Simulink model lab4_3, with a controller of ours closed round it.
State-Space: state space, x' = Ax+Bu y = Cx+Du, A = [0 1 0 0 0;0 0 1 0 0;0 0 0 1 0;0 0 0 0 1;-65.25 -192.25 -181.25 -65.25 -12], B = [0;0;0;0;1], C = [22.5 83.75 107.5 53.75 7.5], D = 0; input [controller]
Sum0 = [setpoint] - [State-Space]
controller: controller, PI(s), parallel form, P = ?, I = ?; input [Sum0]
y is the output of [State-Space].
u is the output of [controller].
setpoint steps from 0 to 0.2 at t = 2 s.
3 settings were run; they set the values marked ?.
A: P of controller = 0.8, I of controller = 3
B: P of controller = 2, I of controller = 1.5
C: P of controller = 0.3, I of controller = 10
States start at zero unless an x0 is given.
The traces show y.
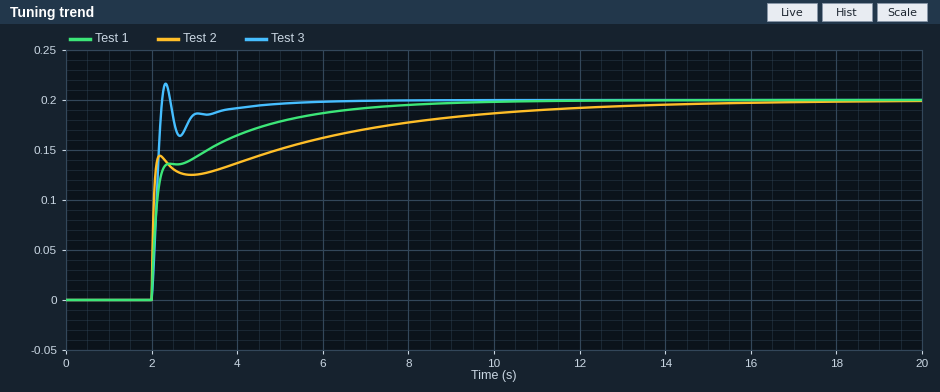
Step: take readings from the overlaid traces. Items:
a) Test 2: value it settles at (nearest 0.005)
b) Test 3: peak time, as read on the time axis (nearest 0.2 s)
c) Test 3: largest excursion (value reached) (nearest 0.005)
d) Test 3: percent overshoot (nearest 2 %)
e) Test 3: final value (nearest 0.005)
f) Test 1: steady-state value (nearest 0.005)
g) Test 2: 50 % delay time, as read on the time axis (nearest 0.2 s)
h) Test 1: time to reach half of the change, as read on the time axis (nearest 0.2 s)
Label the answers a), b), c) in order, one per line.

a) 0.200
b) 2.4 s
c) 0.215
d) 8 %
e) 0.200
f) 0.200
g) 2.0 s
h) 2.2 s
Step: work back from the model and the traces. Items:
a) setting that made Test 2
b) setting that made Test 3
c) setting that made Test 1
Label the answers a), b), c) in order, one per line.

a) B
b) C
c) A
